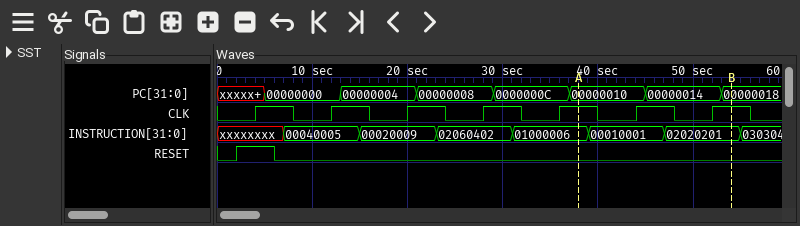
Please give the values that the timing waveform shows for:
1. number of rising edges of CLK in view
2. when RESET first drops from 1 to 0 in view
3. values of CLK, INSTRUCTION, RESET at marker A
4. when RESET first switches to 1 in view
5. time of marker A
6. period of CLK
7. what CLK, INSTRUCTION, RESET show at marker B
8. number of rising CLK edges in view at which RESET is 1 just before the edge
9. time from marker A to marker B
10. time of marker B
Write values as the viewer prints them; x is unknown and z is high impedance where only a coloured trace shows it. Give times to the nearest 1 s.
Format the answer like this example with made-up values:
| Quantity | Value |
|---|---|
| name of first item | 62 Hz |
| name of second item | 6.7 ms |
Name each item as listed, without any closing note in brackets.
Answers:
| Quantity | Value |
|---|---|
| number of rising edges of CLK in view | 7 |
| when RESET first drops from 1 to 0 in view | 6 s |
| values of CLK, INSTRUCTION, RESET at marker A | CLK=1, INSTRUCTION=01000006, RESET=0 |
| when RESET first switches to 1 in view | 2 s |
| time of marker A | 38 s |
| period of CLK | 8 s |
| what CLK, INSTRUCTION, RESET show at marker B | CLK=1, INSTRUCTION=02020201, RESET=0 |
| number of rising CLK edges in view at which RESET is 1 just before the edge | 1 |
| time from marker A to marker B | 16 s |
| time of marker B | 54 s |
